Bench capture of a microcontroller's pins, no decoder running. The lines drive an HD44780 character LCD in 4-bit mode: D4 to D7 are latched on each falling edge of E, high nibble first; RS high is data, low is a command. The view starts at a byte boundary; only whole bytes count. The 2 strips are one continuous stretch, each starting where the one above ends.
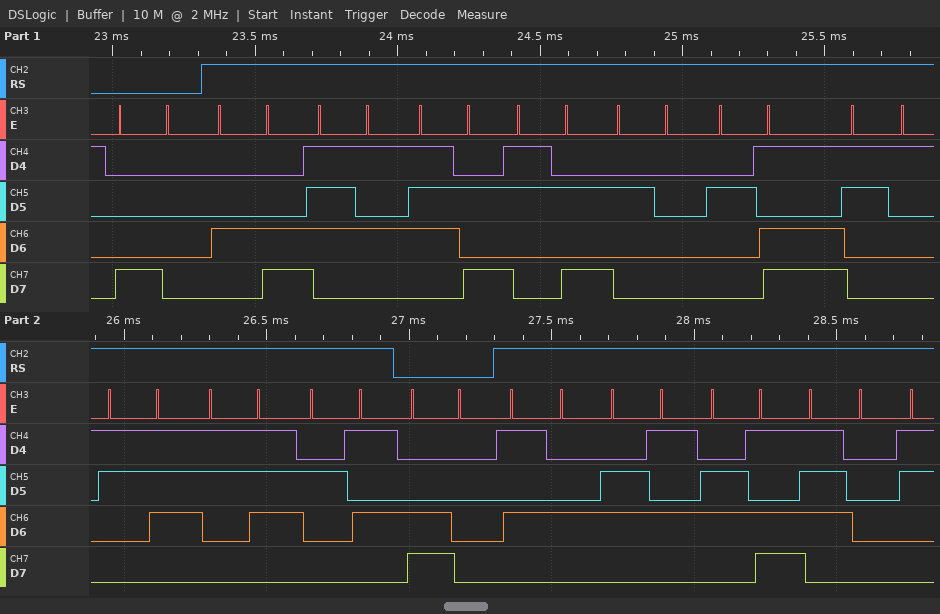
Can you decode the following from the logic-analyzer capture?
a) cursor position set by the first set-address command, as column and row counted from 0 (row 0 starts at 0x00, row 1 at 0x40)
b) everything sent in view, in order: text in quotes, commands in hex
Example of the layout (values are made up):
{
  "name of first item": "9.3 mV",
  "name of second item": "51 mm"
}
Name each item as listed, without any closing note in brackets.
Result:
{
  "cursor position set by the first set-address command, as column and row counted from 0": "column 0, row 0",
  "everything sent in view, in order: text in quotes, commands in hex": "0x80 \"Luz: -177%\" 0xC0 \"Temp\""
}
